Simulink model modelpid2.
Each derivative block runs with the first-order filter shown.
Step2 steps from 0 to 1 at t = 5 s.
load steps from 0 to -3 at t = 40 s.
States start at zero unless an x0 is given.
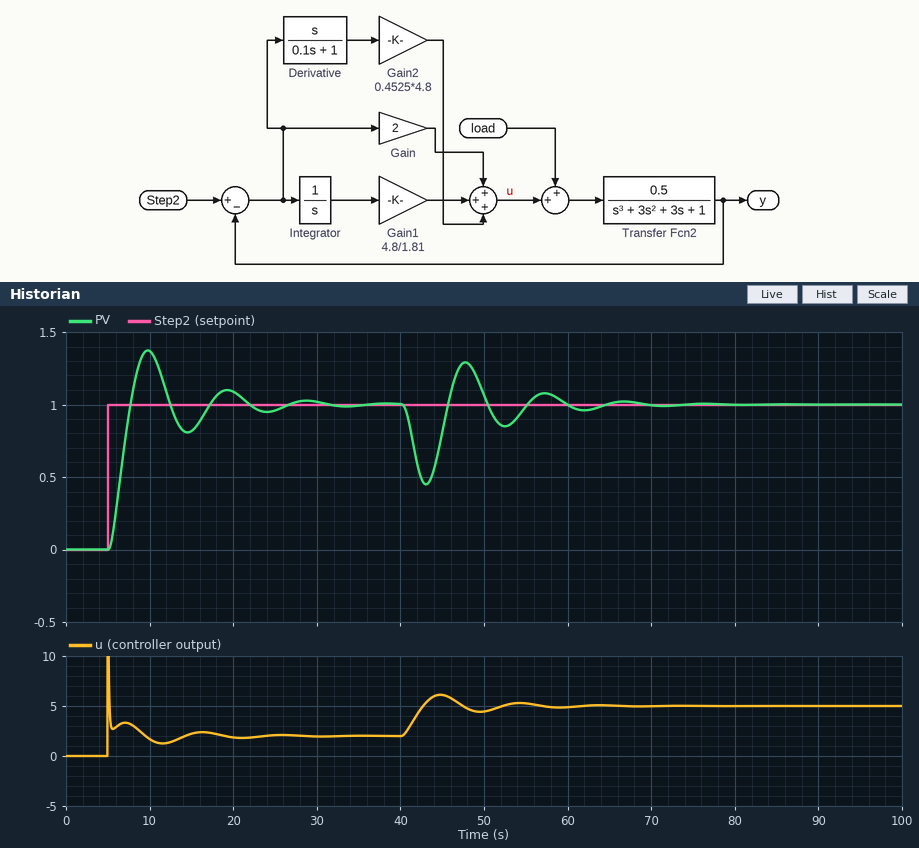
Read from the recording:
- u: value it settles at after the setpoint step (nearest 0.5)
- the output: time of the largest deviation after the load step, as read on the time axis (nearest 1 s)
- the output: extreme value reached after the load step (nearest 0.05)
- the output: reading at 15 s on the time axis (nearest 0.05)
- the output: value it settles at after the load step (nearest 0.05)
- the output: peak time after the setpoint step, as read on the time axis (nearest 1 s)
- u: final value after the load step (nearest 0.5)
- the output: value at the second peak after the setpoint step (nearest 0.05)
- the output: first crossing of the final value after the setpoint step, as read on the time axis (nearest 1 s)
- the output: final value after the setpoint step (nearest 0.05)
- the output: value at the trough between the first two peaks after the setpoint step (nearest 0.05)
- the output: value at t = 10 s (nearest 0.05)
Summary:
2.0
43 s
0.45
0.80
1.00
10 s
5.0
1.10
8 s
1.00
0.80
1.35
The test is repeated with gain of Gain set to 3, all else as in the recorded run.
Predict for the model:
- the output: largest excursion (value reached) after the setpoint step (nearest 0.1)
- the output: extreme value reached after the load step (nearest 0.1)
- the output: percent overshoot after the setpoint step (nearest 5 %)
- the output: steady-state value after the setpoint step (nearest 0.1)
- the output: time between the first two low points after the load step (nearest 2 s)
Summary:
1.3
0.5
30 %
1.0
8 s
